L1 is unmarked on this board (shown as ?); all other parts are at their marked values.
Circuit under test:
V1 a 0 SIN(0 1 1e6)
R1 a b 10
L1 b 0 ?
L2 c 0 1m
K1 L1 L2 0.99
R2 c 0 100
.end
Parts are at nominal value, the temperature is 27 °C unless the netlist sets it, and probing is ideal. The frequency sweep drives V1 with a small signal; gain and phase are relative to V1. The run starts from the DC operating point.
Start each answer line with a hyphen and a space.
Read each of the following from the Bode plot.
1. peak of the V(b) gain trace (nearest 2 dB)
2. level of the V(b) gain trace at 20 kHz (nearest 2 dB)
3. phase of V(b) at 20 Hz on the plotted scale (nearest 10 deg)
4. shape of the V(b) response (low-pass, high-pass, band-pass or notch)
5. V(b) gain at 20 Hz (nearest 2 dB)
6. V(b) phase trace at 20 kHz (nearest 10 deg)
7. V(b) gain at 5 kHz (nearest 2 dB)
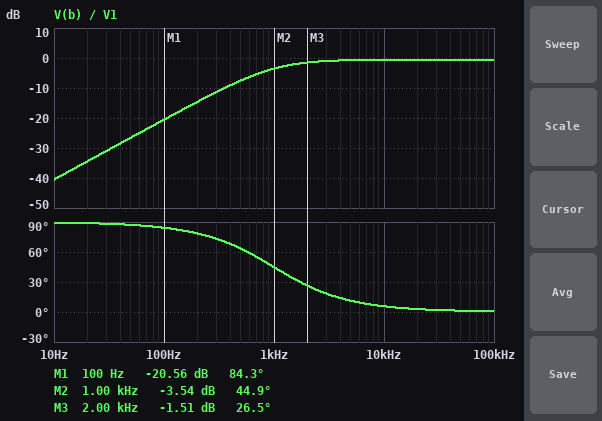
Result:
- 0 dB
- 0 dB
- 90 deg
- high-pass
- -34 dB
- 0 deg
- 0 dB
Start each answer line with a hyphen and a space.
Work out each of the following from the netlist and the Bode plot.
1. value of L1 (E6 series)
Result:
- 1.5 mH
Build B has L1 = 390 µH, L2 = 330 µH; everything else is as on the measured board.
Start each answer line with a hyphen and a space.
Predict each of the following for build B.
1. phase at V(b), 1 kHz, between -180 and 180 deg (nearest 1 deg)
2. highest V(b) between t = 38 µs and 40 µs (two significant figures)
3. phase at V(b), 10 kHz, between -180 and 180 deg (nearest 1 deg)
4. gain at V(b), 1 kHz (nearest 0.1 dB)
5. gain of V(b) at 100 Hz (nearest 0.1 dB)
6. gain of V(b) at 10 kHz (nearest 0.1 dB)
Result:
- 75 deg
- 930 mV
- 21 deg
- -12.5 dB
- -32.2 dB
- -1.3 dB
